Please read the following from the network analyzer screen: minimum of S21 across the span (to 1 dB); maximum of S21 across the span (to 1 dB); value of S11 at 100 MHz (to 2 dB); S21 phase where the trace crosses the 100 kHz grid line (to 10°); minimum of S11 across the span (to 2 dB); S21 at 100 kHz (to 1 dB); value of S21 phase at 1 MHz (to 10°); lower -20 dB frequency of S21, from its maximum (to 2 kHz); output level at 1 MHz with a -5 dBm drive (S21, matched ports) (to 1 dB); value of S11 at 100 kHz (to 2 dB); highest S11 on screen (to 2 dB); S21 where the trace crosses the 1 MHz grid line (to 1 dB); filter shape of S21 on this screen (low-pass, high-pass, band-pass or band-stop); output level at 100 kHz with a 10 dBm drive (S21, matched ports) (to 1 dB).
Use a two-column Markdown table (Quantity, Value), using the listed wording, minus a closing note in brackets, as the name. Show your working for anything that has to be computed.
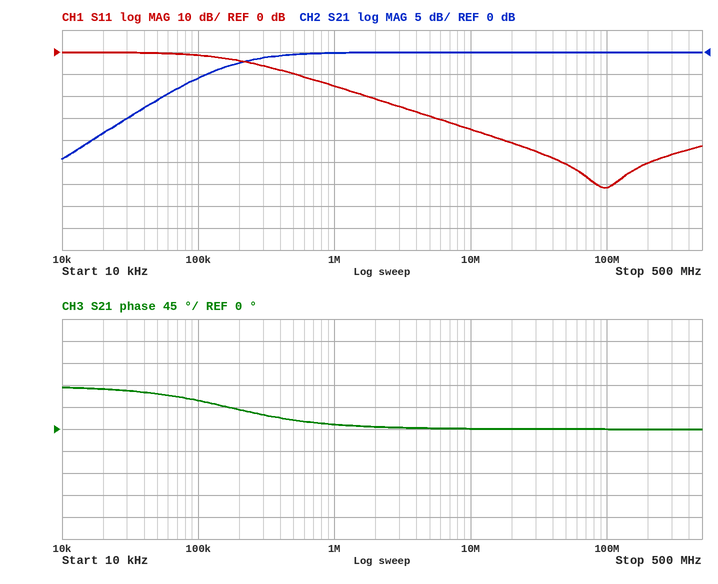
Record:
| Quantity | Value |
|---|---|
| minimum of S21 across the span | -24 dB |
| maximum of S21 across the span | 0 dB |
| value of S11 at 100 MHz | -62 dB |
| S21 phase where the trace crosses the 100 kHz grid line | 60° |
| minimum of S11 across the span | -62 dB |
| S21 at 100 kHz | -6 dB |
| value of S21 phase at 1 MHz | 10° |
| lower -20 dB frequency of S21, from its maximum | 16 kHz |
| output level at 1 MHz with a -5 dBm drive (S21, matched ports) | -5 dBm + (0 dB) = -5 dBm |
| value of S11 at 100 kHz | -2 dB |
| highest S11 on screen | 0 dB |
| S21 where the trace crosses the 1 MHz grid line | 0 dB |
| filter shape of S21 on this screen | high-pass |
| output level at 100 kHz with a 10 dBm drive (S21, matched ports) | 10 dBm + (-6 dB) = 4 dBm |
